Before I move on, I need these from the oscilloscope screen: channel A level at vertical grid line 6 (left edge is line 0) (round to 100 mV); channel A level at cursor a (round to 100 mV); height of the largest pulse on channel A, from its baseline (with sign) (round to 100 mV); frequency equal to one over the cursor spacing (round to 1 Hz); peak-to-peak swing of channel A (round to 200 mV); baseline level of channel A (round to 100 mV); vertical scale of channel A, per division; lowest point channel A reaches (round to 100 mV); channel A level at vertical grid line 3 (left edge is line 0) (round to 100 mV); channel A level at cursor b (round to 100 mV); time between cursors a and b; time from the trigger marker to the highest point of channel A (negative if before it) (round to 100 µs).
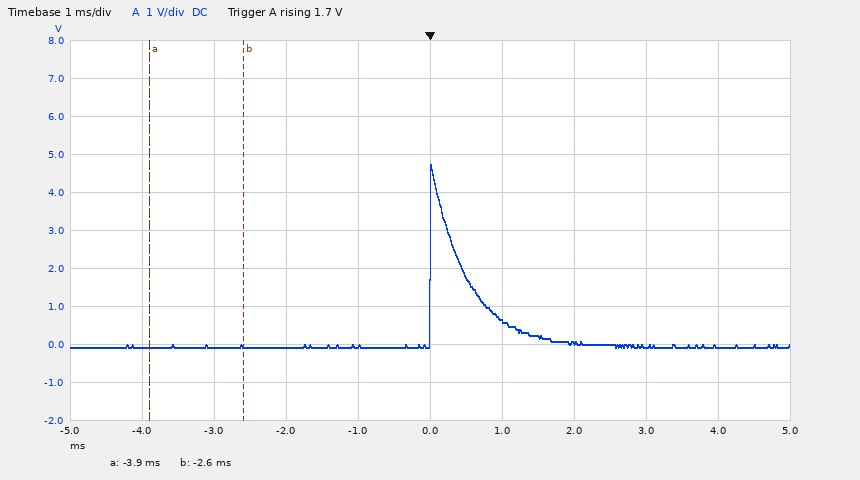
600 mV
-100 mV
+4.8 V
769 Hz
4.8 V
-100 mV
1 V
-100 mV
-100 mV
0.0 V
1.3 ms
0.0 ms
